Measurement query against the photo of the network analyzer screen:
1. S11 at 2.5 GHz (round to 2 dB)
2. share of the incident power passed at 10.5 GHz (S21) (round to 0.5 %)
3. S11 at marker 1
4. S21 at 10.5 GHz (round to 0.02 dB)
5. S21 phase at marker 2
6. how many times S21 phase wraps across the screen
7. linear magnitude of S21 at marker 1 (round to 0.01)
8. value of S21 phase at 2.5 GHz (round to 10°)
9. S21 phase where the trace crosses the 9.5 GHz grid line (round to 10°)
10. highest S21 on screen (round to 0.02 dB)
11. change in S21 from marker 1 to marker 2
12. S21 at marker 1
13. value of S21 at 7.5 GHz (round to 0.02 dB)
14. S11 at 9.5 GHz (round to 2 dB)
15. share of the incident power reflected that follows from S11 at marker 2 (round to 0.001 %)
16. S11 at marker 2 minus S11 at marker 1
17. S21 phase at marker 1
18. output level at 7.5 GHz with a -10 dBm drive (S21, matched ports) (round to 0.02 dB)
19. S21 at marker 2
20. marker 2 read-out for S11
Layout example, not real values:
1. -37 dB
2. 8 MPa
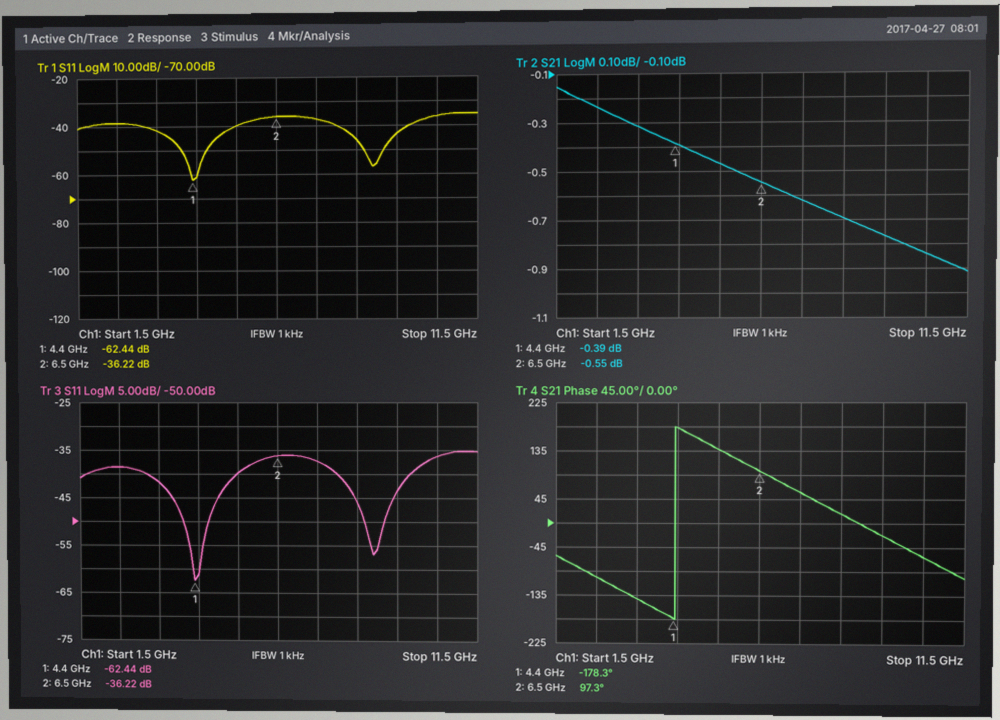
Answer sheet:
1. -38 dB
2. 82.5 %
3. -62.44 dB
4. -0.84 dB
5. 97.3°
6. 1
7. 0.96
8. -100°
9. -20°
10. -0.16 dB
11. -0.16 dB
12. -0.39 dB
13. -0.62 dB
14. -44 dB
15. 0.024 %
16. 26.22 dB
17. -178.3°
18. -10.62 dBm
19. -0.55 dB
20. -36.22 dB
